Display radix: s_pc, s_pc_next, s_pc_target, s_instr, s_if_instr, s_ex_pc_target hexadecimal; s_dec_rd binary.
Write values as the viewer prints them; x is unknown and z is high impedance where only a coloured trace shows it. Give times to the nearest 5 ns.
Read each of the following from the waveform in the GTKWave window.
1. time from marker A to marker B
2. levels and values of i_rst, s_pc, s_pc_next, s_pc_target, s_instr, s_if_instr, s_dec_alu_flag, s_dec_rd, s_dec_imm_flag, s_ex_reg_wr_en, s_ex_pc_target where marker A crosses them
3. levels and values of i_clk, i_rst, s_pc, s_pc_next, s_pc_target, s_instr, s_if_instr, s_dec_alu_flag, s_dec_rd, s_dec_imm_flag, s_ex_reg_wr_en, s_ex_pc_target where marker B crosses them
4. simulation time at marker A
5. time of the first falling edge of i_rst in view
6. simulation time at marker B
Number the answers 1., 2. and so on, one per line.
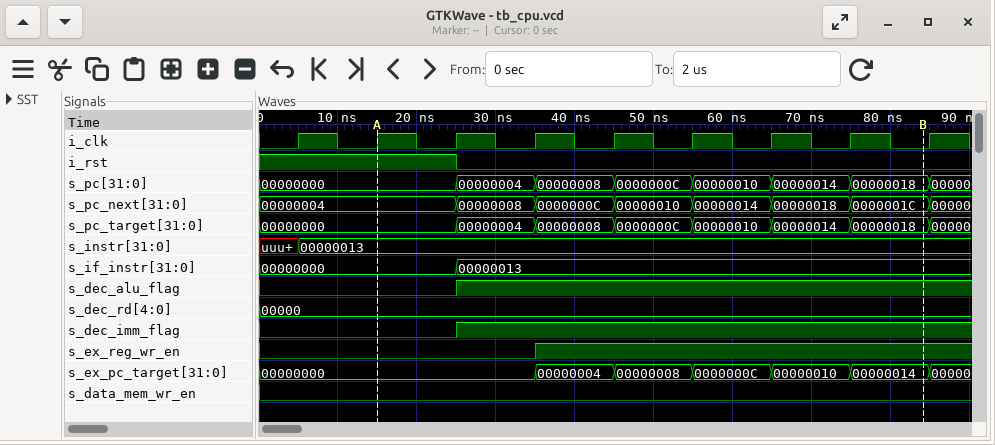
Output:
1. 70 ns
2. i_rst=1, s_pc=00000000, s_pc_next=00000004, s_pc_target=00000000, s_instr=00000013, s_if_instr=00000000, s_dec_alu_flag=0, s_dec_rd=00000, s_dec_imm_flag=0, s_ex_reg_wr_en=0, s_ex_pc_target=00000000
3. i_clk=0, i_rst=0, s_pc=00000018, s_pc_next=0000001C, s_pc_target=00000018, s_instr=00000013, s_if_instr=00000013, s_dec_alu_flag=1, s_dec_rd=00000, s_dec_imm_flag=1, s_ex_reg_wr_en=1, s_ex_pc_target=00000014
4. 15 ns
5. 25 ns
6. 85 ns
